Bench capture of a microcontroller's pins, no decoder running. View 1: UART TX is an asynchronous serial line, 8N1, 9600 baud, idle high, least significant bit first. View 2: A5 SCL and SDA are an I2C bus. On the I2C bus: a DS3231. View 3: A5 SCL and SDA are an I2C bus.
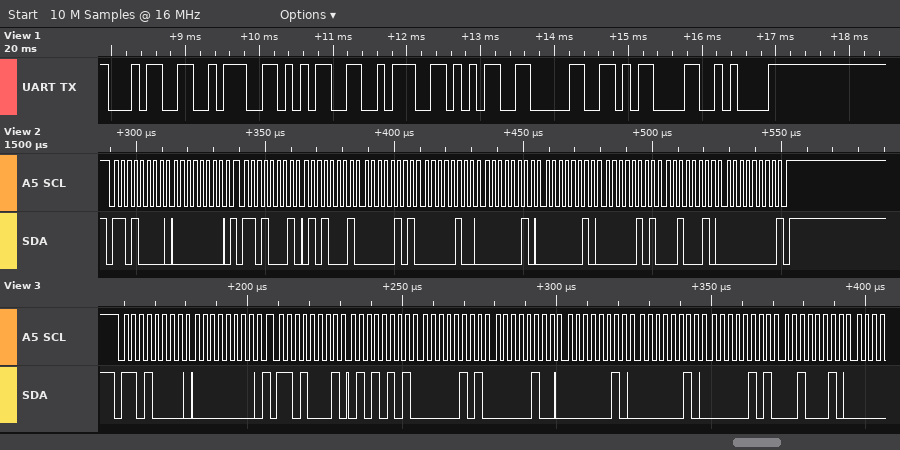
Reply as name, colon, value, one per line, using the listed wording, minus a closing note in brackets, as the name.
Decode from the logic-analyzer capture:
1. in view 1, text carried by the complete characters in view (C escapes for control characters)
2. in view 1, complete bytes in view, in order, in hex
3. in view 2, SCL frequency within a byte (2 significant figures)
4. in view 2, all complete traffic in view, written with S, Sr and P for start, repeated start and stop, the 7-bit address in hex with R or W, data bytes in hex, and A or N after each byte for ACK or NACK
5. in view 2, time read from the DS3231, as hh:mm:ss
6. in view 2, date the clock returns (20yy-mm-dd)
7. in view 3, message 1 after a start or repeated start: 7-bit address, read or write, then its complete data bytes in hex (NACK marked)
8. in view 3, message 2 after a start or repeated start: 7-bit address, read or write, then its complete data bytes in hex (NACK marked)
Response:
in view 1, text carried by the complete characters in view: "4:5:50\r\n"
in view 1, complete bytes in view, in order, in hex: 34 3A 35 3A 35 30 0D 0A
in view 2, SCL frequency within a byte: 400 kHz
in view 2, all complete traffic in view, written with S, Sr and P for start, repeated start and stop, the 7-bit address in hex with R or W, data bytes in hex, and A or N after each byte for ACK or NACK: S 68W A 00 A Sr 68R A 51 A 05 A 04 A 02 A 02 A 05 A 22 A 00 N P
in view 2, time read from the DS3231, as hh:mm:ss: 04:05:51
in view 2, date the clock returns: 2022-05-02
in view 3, message 1 after a start or repeated start: 7-bit address, read or write, then its complete data bytes in hex: 0x68 write: 00
in view 3, message 2 after a start or repeated start: 7-bit address, read or write, then its complete data bytes in hex: 0x68 read: 55 05 04 02 02 05 22
